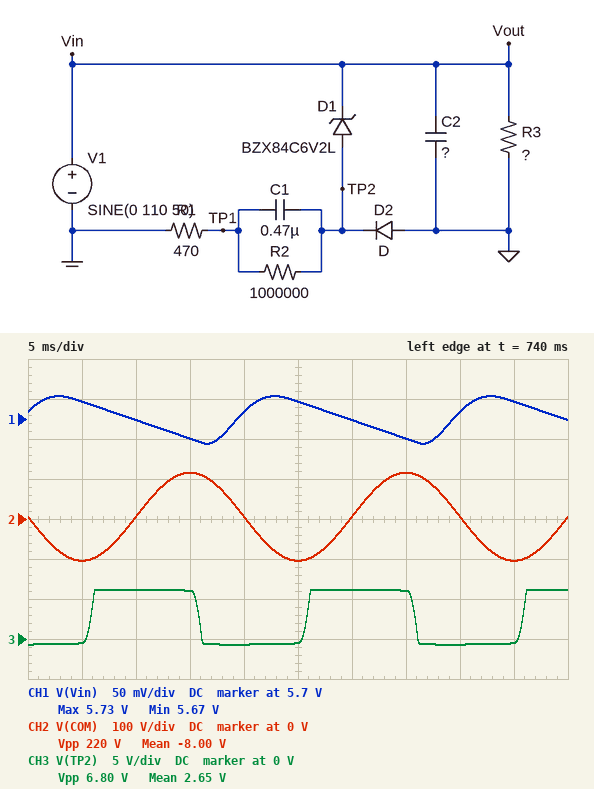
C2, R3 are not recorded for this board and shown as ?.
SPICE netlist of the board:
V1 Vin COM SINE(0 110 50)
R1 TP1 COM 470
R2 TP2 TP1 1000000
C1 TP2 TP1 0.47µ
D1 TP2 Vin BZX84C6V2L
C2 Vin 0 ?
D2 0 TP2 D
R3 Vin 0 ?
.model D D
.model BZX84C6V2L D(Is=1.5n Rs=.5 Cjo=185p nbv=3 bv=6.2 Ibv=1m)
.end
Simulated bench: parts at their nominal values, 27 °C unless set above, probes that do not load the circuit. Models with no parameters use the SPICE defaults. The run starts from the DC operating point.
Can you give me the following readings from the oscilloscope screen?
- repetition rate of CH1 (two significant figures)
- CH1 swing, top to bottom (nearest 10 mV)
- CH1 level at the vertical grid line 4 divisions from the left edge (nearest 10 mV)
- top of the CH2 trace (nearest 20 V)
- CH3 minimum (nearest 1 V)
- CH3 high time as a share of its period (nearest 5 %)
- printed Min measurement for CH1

50 Hz
60 mV
5.71 V
120 V
-1 V
50 %
5.67 V
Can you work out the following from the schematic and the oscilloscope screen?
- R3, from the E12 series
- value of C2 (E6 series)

5.6 kΩ
220 µF
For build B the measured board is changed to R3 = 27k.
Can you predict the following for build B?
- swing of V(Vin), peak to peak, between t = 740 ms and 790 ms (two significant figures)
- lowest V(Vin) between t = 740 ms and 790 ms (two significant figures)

13 mV
5.8 V
